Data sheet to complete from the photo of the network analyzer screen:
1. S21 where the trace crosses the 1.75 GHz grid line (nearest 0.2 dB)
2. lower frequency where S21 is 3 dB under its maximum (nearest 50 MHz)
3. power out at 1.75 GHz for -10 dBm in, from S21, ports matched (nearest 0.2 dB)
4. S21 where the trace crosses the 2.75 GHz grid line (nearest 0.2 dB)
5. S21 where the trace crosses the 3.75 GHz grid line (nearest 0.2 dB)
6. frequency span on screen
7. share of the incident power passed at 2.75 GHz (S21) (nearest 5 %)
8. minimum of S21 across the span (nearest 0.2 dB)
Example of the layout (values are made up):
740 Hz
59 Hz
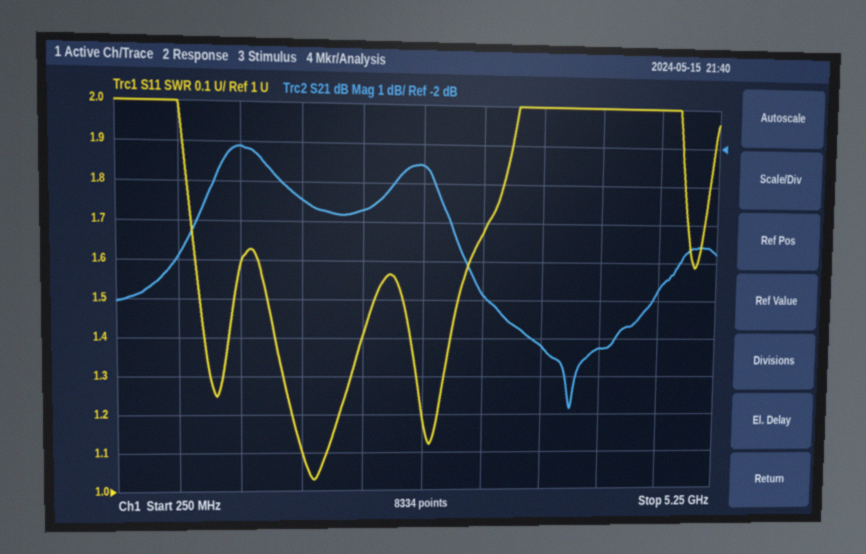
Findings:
-3.4 dB
700 MHz
-13.4 dBm
-2.6 dB
-7.2 dB
5 GHz
55 %
-8.8 dB
